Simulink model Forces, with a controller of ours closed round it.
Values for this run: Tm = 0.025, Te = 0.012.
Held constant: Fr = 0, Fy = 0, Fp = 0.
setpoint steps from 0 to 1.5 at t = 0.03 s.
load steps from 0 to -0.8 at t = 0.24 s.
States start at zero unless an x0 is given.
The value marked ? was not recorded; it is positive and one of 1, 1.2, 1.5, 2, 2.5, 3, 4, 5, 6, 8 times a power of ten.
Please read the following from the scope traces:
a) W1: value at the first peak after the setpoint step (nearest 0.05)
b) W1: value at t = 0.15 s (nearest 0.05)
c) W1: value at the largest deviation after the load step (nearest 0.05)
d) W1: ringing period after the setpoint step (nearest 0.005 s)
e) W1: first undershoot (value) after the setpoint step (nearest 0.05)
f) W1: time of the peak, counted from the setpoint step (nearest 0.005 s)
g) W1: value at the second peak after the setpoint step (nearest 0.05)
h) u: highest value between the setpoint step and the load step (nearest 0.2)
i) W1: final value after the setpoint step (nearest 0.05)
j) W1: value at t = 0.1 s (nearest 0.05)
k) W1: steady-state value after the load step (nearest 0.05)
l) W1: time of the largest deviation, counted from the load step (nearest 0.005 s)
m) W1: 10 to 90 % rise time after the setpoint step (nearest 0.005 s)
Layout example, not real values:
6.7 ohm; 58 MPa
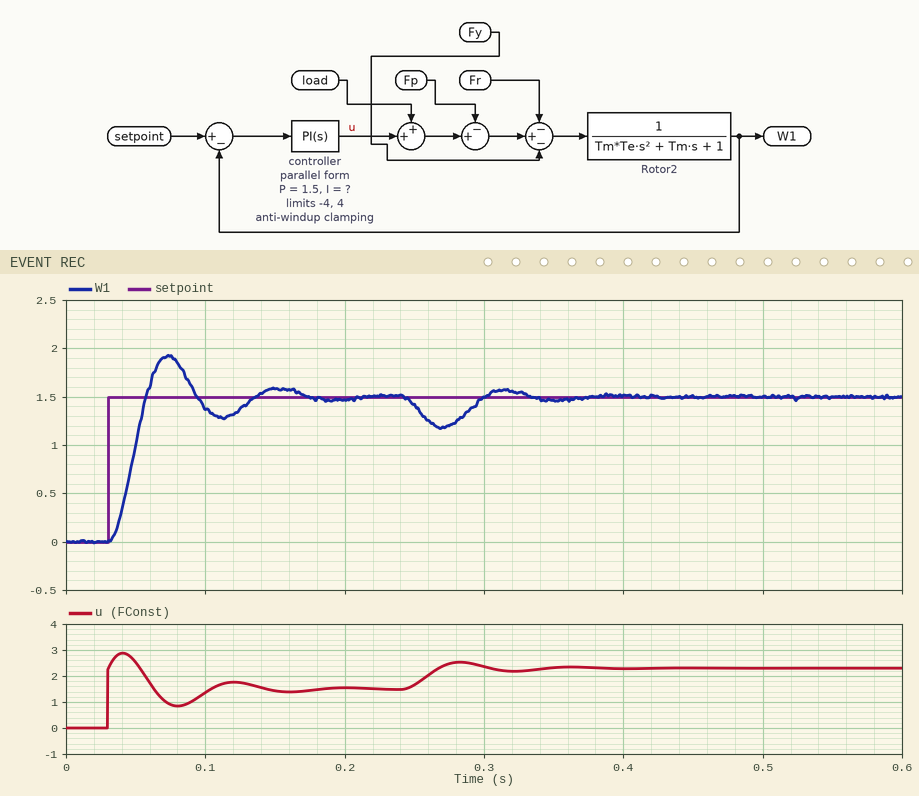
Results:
1.90; 1.60; 1.20; 0.080 s; 1.30; 0.045 s; 1.60; 2.8; 1.50; 1.40; 1.50; 0.030 s; 0.020 s
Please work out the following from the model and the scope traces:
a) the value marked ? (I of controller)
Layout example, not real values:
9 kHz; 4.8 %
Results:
80
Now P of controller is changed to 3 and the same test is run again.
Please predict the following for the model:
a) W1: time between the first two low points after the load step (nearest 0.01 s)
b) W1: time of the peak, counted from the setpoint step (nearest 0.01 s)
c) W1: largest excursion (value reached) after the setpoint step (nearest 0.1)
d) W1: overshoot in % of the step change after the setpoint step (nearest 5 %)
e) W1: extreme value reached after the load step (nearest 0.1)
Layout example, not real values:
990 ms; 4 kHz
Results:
0.06 s; 0.03 s; 1.7; 15 %; 1.3
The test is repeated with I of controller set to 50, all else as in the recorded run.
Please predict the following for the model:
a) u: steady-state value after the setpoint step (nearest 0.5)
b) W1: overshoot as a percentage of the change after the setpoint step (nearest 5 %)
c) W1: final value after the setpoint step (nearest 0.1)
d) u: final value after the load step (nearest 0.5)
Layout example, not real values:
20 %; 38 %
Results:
1.5; 10 %; 1.5; 2.5
